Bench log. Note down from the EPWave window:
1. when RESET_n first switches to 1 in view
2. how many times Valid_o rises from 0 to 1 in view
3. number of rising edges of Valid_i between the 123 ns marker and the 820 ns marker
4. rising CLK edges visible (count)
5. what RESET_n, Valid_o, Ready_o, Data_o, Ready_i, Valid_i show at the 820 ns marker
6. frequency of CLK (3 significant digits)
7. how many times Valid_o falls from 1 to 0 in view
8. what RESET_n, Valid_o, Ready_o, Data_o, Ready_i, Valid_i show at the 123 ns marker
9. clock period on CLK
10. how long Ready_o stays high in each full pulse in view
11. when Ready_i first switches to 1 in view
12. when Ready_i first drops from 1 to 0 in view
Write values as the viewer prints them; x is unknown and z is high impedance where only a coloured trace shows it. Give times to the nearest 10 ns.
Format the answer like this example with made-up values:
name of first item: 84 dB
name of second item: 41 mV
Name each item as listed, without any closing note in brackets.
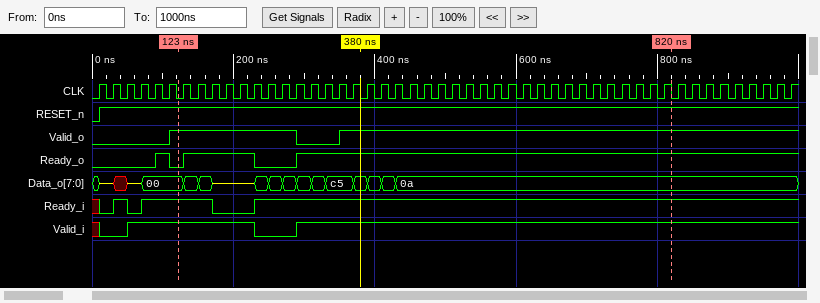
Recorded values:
when RESET_n first switches to 1 in view: 10 ns
how many times Valid_o rises from 0 to 1 in view: 2
number of rising edges of Valid_i between the 123 ns marker and the 820 ns marker: 1
rising CLK edges visible: 50
what RESET_n, Valid_o, Ready_o, Data_o, Ready_i, Valid_i show at the 820 ns marker: RESET_n=1, Valid_o=1, Ready_o=1, Data_o=0a, Ready_i=1, Valid_i=1
frequency of CLK: 50.0 MHz
how many times Valid_o falls from 1 to 0 in view: 1
what RESET_n, Valid_o, Ready_o, Data_o, Ready_i, Valid_i show at the 123 ns marker: RESET_n=1, Valid_o=1, Ready_o=0, Data_o=00, Ready_i=1, Valid_i=1
clock period on CLK: 20 ns
how long Ready_o stays high in each full pulse in view: 20 ns, 100 ns
when Ready_i first switches to 1 in view: 30 ns
when Ready_i first drops from 1 to 0 in view: 50 ns
